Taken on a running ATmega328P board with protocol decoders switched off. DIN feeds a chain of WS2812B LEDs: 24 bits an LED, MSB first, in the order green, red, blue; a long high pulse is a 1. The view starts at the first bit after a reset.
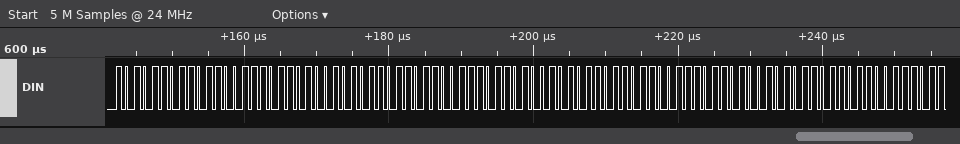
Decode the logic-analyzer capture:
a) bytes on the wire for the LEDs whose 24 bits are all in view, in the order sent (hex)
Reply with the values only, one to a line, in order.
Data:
AD B3 B4 AD B3 B4 AD B3 B4
